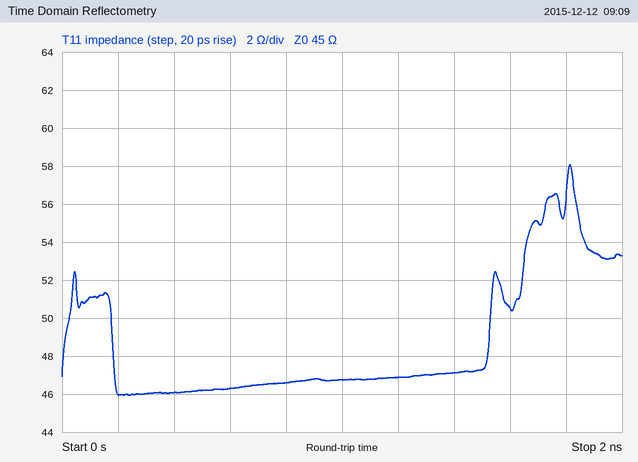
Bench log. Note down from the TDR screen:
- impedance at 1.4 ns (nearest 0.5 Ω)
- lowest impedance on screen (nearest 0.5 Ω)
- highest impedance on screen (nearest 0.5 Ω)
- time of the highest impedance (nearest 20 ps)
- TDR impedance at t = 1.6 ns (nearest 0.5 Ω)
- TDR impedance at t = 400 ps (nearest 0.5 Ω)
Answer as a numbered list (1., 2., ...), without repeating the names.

1. 47.0 Ω
2. 46.0 Ω
3. 58.0 Ω
4. 1.82 ns
5. 50.5 Ω
6. 46.0 Ω
